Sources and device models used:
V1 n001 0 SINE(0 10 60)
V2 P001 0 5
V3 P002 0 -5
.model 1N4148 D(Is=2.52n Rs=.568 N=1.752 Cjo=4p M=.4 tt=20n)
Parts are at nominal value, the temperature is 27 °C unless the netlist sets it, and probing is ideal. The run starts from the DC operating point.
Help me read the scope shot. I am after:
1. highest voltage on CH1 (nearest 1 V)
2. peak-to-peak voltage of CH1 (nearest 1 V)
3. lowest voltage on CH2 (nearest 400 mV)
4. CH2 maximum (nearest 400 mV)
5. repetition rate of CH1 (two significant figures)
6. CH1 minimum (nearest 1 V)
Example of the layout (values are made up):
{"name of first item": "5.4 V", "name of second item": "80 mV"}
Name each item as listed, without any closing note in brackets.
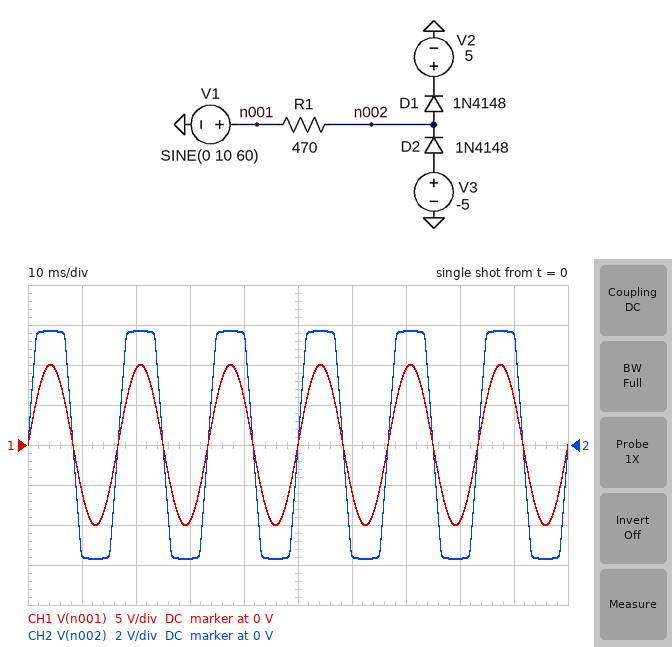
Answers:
{"highest voltage on CH1": "10 V", "peak-to-peak voltage of CH1": "20 V", "lowest voltage on CH2": "-5.6 V", "CH2 maximum": "5.6 V", "repetition rate of CH1": "60 Hz", "CH1 minimum": "-10 V"}
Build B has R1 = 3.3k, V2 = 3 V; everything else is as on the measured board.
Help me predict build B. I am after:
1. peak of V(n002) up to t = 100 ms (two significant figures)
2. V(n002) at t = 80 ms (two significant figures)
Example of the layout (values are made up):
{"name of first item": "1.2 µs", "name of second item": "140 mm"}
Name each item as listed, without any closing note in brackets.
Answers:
{"peak of V(n002) up to t = 100 ms": "3.6 V", "V(n002) at t = 80 ms": "-5.6 V"}
